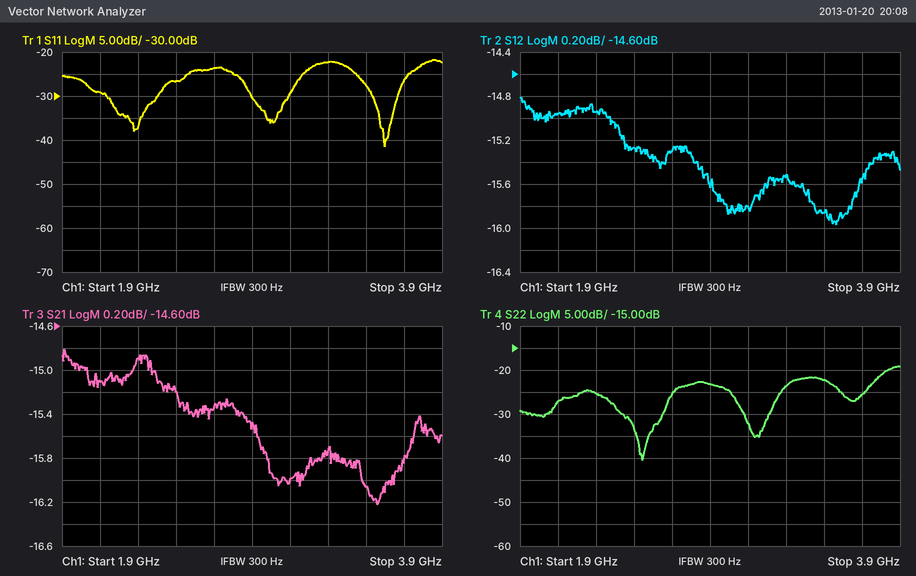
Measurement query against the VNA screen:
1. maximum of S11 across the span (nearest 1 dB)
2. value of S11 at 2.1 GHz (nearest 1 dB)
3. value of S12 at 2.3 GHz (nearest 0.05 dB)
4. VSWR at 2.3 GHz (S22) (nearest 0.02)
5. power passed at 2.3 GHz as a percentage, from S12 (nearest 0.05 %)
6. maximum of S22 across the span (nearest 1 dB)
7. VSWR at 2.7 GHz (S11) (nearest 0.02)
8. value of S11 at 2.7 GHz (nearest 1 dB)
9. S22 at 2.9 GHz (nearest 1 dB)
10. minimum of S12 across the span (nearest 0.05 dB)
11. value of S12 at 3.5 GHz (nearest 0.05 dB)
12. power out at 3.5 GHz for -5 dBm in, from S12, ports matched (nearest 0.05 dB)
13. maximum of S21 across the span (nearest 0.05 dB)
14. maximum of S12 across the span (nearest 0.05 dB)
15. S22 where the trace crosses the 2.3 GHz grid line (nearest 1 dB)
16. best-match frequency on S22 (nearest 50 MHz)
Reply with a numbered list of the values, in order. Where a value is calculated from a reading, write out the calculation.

1. -22 dB
2. -29 dB
3. -14.95 dB
4. |Γ| = 10^(-25/20) = 0.0562; VSWR = (1 + 0.0562)/(1 − 0.0562) ≈ 1.12
5. 10^(-14.95/10) ≈ 3.20 %
6. -19 dB
7. |Γ| = 10^(-24/20) = 0.0631; VSWR = (1 + 0.0631)/(1 − 0.0631) ≈ 1.13, so 1.14 to the nearest 0.02
8. -24 dB
9. -23 dB
10. -15.95 dB
11. -15.85 dB
12. -5 dBm + (-15.85 dB) = -20.85 dBm
13. -14.80 dB
14. -14.80 dB
15. -25 dB
16. 2.55 GHz
